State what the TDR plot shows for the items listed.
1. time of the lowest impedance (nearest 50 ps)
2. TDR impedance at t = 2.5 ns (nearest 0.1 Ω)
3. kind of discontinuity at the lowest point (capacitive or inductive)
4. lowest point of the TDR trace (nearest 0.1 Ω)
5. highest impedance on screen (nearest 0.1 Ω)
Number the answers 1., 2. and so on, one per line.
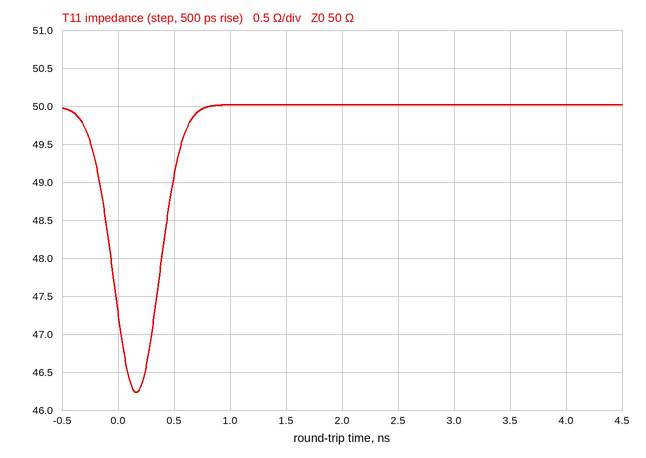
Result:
1. 150 ps
2. 50.0 Ω
3. capacitive
4. 46.2 Ω
5. 50.0 Ω
